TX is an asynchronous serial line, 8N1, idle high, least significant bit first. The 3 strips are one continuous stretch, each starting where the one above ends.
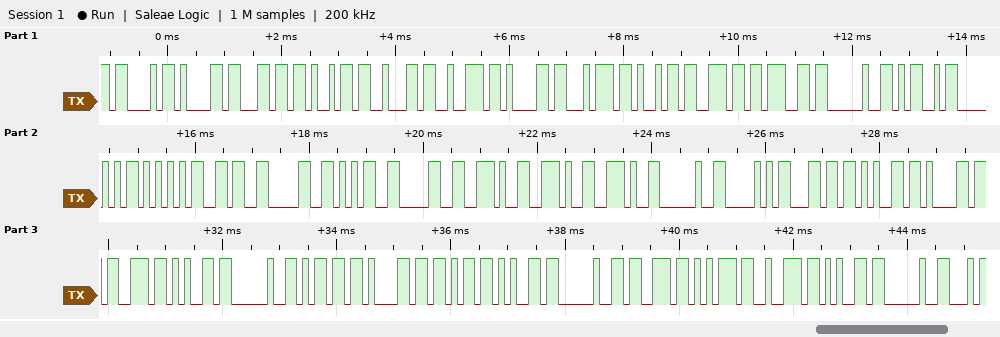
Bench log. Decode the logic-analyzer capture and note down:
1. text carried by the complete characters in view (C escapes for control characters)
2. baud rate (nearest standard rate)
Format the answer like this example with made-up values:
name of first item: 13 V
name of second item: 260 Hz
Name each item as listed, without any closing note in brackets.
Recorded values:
text carried by the complete characters in view: "Calibrating MPU6050... Please make sure "
baud rate: 9600 baud
